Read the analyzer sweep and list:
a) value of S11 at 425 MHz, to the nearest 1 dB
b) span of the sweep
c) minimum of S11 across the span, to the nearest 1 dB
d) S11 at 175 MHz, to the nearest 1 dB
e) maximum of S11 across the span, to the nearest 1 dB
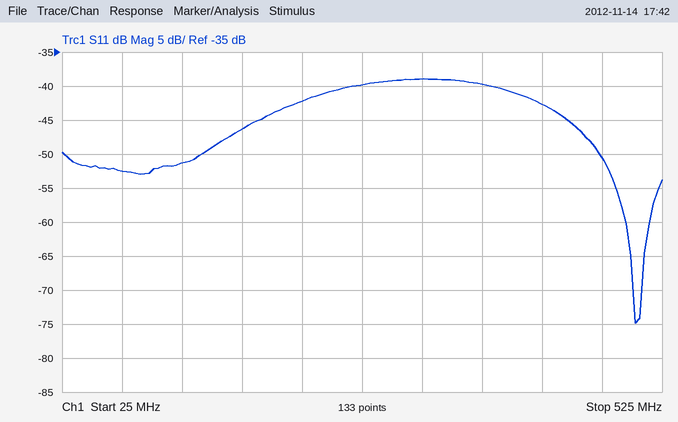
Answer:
-43 dB
500 MHz
-75 dB
-46 dB
-39 dB
